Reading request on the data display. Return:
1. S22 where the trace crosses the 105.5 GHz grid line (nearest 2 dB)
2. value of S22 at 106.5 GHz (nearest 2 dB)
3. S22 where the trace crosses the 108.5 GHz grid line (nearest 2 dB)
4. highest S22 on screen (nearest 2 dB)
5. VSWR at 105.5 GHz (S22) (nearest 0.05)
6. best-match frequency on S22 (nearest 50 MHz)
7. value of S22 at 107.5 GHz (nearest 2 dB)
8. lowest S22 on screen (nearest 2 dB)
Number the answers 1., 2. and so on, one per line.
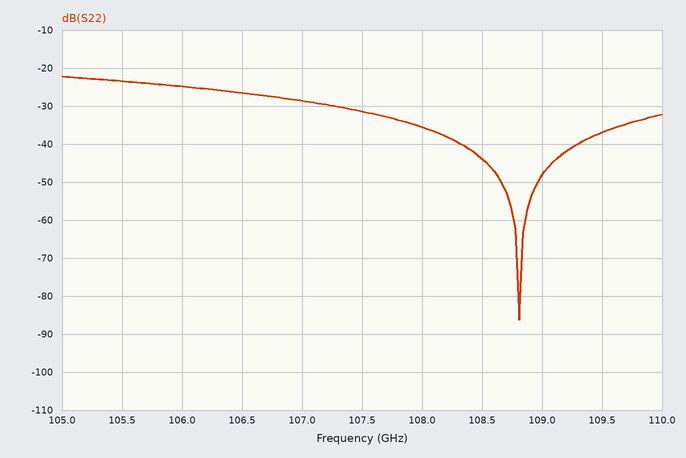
1. -24 dB
2. -26 dB
3. -44 dB
4. -22 dB
5. 1.15
6. 108.80 GHz
7. -32 dB
8. -86 dB
